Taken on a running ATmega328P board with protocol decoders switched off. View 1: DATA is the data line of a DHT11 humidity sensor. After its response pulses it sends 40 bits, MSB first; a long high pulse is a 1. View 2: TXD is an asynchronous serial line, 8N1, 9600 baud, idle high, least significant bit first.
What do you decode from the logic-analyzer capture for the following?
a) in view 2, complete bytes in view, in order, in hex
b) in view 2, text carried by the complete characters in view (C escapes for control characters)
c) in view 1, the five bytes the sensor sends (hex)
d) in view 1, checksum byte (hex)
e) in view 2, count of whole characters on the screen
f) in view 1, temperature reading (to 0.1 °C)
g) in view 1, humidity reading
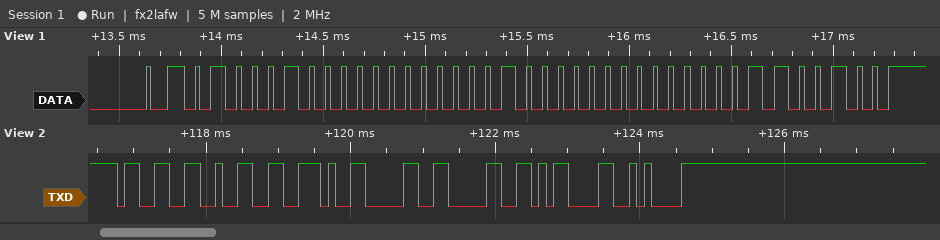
33 32 2E 30 30 0D 0A
"32.00\r\n"
44 00 20 00 64
0x64
7
32.0 °C
68 %
